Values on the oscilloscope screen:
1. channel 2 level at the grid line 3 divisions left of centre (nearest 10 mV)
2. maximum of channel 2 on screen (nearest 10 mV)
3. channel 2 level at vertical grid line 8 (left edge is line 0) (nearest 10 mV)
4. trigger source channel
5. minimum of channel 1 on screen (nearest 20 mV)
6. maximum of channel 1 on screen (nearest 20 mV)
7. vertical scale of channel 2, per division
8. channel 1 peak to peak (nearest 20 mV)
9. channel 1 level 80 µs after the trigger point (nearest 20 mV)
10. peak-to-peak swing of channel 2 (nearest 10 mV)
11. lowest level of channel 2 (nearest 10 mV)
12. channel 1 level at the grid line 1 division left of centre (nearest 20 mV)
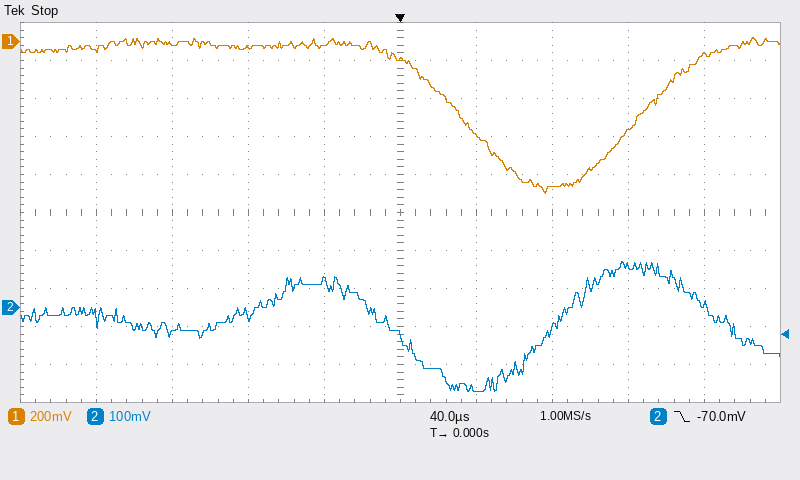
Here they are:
-70 mV
120 mV
110 mV
channel 2
-800 mV
20 mV
100 mV
820 mV
-760 mV
340 mV
-220 mV
-20 mV
